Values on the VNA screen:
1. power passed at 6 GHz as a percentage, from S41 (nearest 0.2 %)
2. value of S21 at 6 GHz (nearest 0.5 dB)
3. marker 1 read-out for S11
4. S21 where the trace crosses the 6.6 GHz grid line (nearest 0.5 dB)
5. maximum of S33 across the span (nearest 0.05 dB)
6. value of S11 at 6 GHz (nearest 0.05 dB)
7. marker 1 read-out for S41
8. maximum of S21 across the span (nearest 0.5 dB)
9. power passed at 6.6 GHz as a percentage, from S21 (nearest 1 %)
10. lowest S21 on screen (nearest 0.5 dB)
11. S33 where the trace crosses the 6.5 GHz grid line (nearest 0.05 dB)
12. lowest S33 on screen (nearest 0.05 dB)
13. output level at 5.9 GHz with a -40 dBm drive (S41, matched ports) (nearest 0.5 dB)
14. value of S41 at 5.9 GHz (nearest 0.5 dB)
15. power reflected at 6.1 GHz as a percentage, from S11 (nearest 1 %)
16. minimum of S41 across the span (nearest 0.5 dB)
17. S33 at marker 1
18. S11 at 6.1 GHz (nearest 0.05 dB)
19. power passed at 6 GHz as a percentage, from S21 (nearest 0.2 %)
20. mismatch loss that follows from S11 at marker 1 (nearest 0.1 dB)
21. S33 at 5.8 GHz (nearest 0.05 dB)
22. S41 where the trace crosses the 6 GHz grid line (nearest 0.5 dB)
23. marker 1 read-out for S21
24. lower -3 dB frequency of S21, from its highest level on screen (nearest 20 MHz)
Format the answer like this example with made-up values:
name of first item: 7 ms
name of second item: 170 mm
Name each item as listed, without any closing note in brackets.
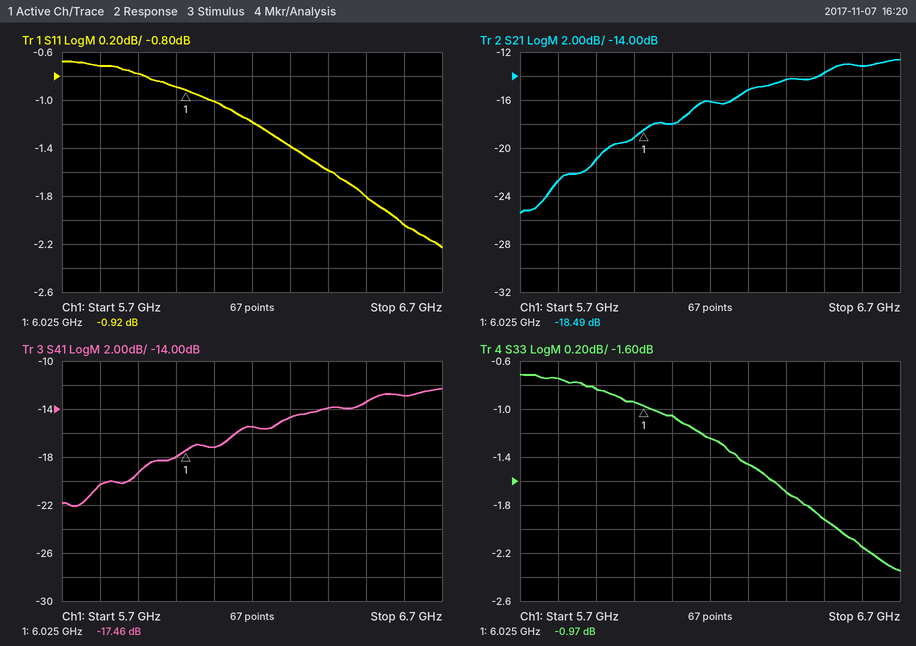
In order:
power passed at 6 GHz as a percentage, from S41: 1.6 %
value of S21 at 6 GHz: -19.0 dB
marker 1 read-out for S11: -0.92 dB
S21 where the trace crosses the 6.6 GHz grid line: -13.0 dB
maximum of S33 across the span: -0.70 dB
value of S11 at 6 GHz: -0.90 dB
marker 1 read-out for S41: -17.46 dB
maximum of S21 across the span: -12.5 dB
power passed at 6.6 GHz as a percentage, from S21: 5 %
lowest S21 on screen: -25.5 dB
S33 where the trace crosses the 6.5 GHz grid line: -1.90 dB
lowest S33 on screen: -2.35 dB
output level at 5.9 GHz with a -40 dBm drive (S41, matched ports): -59.5 dBm
value of S41 at 5.9 GHz: -19.5 dB
power reflected at 6.1 GHz as a percentage, from S11: 79 %
minimum of S41 across the span: -22.0 dB
S33 at marker 1: -0.97 dB
S11 at 6.1 GHz: -1.00 dB
power passed at 6 GHz as a percentage, from S21: 1.2 %
mismatch loss that follows from S11 at marker 1: 7.2 dB
S33 at 5.8 GHz: -0.75 dB
S41 where the trace crosses the 6 GHz grid line: -18.0 dB
marker 1 read-out for S21: -18.49 dB
lower -3 dB frequency of S21, from its highest level on screen: 6.28 GHz
